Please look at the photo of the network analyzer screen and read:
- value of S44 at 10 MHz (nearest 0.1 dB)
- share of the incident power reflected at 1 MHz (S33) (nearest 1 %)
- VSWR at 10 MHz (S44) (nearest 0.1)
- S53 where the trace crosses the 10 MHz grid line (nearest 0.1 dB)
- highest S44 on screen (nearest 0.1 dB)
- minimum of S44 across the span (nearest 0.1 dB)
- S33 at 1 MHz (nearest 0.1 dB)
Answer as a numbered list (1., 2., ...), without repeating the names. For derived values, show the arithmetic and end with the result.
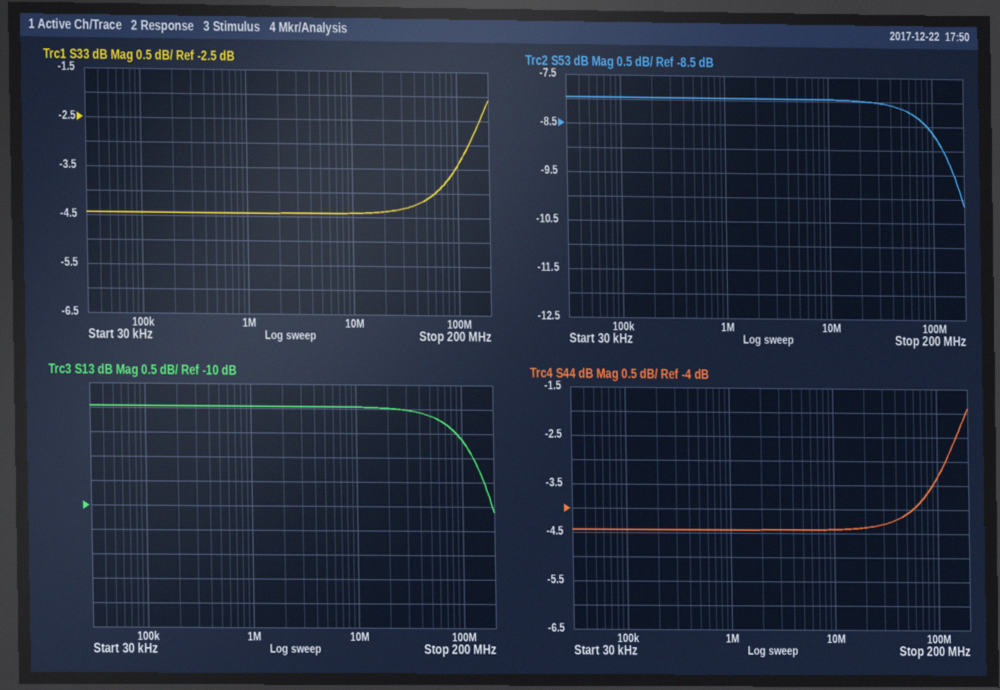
1. -4.4 dB
2. 10^(-4.4/10) ≈ 36 %
3. |Γ| = 10^(-4.4/20) = 0.6026; VSWR = (1 + 0.6026)/(1 − 0.6026) ≈ 4.0
4. -8.0 dB
5. -1.9 dB
6. -4.4 dB
7. -4.4 dB
